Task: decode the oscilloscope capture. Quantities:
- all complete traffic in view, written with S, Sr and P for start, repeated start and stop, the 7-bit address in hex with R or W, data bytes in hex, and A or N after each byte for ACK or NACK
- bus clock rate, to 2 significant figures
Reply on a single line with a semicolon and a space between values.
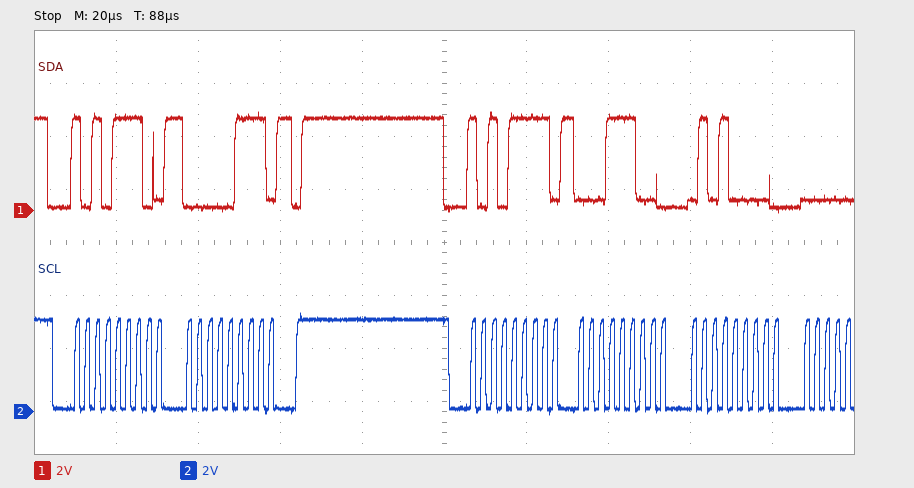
S 57W A 07 A P S 57R A 1C A 50 A; 400 kHz
